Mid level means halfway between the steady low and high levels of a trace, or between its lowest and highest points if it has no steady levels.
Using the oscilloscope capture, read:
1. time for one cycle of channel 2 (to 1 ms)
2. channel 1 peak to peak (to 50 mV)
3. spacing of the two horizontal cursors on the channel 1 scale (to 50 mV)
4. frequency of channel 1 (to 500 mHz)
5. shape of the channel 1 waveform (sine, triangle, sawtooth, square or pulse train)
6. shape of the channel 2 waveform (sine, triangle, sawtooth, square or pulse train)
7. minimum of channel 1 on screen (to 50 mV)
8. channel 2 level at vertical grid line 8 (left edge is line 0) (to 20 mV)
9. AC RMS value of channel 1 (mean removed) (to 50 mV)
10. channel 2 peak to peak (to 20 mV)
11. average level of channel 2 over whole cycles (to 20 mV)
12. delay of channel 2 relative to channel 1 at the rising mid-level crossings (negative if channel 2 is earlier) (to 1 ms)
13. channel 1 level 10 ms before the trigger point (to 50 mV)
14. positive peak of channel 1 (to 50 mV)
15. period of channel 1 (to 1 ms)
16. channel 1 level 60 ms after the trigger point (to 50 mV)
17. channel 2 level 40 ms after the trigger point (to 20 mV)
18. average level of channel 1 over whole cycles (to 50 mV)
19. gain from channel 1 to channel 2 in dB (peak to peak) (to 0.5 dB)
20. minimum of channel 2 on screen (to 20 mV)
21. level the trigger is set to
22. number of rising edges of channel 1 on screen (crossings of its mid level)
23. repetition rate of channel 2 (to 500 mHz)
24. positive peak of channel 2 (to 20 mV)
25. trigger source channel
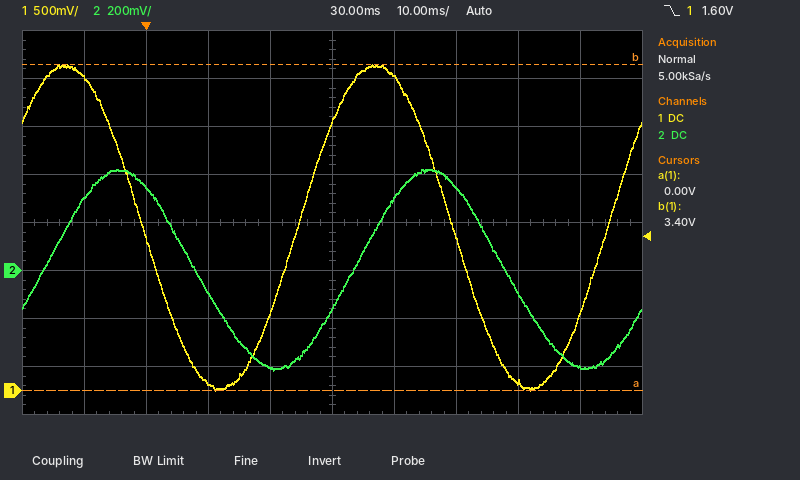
50 ms
3.40 V
3.40 V
20.0 Hz
sine
sine
0 mV
-100 mV
1.20 V
840 mV
0 mV
+9 ms
3.25 V
3.40 V
50 ms
100 mV
300 mV
1.70 V
-12.0 dB
-420 mV
1.60 V
2
20.0 Hz
420 mV
channel 1
